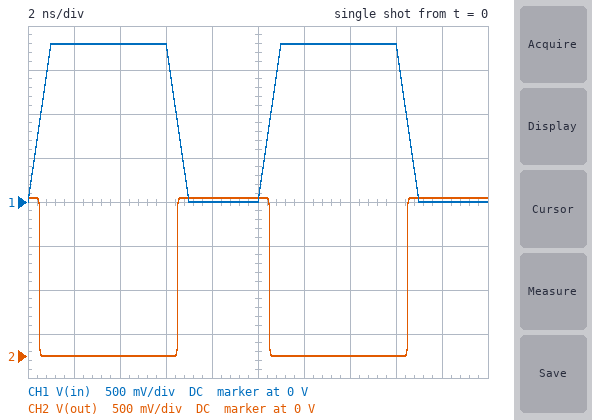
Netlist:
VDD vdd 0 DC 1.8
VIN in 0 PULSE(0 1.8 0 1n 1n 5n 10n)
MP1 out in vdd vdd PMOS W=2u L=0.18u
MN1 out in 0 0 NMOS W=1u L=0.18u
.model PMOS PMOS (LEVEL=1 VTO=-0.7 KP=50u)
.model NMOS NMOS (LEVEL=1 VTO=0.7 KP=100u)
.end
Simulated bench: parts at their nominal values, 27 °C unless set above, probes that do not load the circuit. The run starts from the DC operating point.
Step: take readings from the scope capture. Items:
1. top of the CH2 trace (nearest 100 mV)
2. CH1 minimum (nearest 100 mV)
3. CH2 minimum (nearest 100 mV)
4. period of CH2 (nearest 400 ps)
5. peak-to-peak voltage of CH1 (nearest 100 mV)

1.8 V
0 V
0 V
10.0 ns
1.8 V
